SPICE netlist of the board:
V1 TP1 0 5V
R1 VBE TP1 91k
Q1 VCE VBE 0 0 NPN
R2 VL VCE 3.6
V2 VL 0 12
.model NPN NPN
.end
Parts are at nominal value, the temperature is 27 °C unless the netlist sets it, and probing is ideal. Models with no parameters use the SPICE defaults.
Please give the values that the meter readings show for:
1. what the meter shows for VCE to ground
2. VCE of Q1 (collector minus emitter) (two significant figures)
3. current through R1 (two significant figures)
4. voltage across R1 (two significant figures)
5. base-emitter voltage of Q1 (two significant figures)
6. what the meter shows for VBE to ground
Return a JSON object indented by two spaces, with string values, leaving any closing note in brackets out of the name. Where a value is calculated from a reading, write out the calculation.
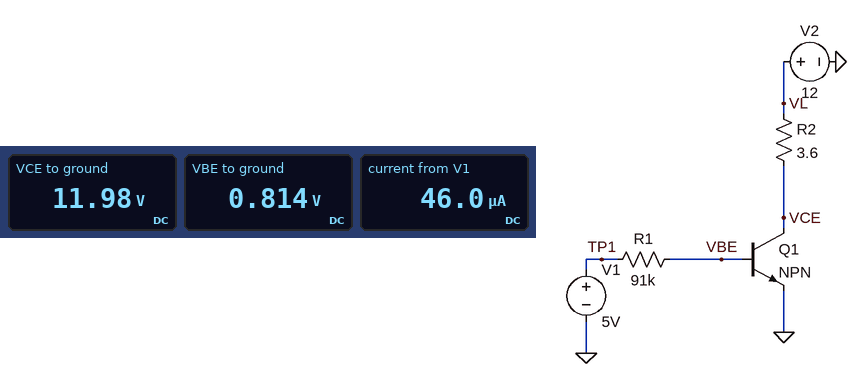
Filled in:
{
  "what the meter shows for VCE to ground": "11.98 V",
  "VCE of Q1 (collector minus emitter)": "11.98 V = 12 V",
  "current through R1": "(5 V - 814 mV) / 91 kΩ = 46 µA",
  "voltage across R1": "5 V - 814 mV = 4.2 V",
  "base-emitter voltage of Q1": "814 mV = 810 mV",
  "what the meter shows for VBE to ground": "0.814 V"
}
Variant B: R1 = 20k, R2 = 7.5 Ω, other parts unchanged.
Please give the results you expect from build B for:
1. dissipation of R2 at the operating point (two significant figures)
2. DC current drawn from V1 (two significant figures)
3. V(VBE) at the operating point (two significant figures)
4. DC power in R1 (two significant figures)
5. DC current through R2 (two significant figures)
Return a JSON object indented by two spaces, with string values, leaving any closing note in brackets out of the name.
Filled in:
{
  "dissipation of R2 at the operating point": "3.2 mW",
  "DC current drawn from V1": "210 µA",
  "V(VBE) at the operating point": "850 mV",
  "DC power in R1": "860 µW",
  "DC current through R2": "21 mA"
}
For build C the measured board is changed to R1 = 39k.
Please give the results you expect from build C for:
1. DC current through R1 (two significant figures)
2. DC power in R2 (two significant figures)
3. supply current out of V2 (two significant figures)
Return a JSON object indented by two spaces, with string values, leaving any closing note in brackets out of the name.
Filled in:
{
  "DC current through R1": "110 µA",
  "DC power in R2": "410 µW",
  "supply current out of V2": "11 mA"
}
